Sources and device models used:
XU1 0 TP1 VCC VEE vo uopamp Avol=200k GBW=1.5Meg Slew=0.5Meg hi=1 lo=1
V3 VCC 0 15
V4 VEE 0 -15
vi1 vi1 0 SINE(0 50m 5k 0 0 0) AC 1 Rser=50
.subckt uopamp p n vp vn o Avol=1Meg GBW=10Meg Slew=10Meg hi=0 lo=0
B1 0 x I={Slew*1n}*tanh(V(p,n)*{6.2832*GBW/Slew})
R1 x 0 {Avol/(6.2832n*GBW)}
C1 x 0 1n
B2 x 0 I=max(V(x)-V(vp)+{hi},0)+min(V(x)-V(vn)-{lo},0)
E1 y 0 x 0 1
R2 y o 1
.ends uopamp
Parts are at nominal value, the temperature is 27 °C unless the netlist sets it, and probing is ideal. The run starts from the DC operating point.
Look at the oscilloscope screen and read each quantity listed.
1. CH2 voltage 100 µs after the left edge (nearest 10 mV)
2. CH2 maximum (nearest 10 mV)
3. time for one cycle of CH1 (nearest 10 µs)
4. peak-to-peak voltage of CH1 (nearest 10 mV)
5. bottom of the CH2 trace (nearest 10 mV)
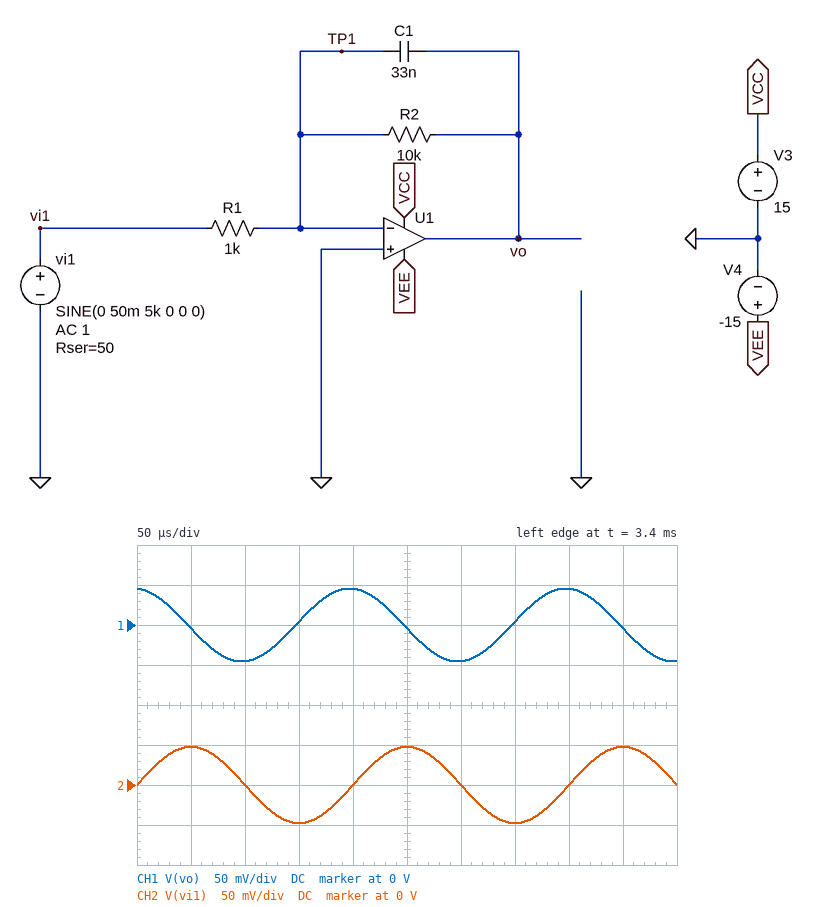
0 V
50 mV
200 µs
90 mV
-50 mV
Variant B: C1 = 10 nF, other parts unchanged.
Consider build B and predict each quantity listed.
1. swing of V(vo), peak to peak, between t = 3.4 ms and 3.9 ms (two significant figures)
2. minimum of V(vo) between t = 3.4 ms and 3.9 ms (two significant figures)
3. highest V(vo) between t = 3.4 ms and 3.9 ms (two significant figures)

290 mV
-140 mV
140 mV
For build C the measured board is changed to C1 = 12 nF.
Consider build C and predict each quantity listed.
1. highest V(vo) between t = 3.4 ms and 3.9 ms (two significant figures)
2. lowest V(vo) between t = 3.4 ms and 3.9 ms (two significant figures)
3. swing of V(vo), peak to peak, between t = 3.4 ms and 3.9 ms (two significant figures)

120 mV
-120 mV
240 mV
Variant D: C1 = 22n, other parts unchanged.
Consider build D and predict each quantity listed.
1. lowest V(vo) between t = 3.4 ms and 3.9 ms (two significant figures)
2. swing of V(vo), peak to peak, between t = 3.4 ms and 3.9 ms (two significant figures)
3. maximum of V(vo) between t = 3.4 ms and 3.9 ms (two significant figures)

-68 mV
140 mV
68 mV
